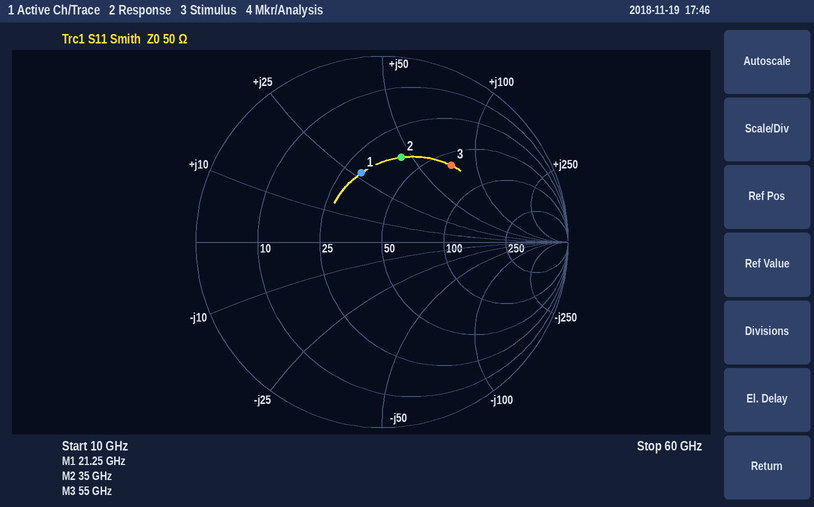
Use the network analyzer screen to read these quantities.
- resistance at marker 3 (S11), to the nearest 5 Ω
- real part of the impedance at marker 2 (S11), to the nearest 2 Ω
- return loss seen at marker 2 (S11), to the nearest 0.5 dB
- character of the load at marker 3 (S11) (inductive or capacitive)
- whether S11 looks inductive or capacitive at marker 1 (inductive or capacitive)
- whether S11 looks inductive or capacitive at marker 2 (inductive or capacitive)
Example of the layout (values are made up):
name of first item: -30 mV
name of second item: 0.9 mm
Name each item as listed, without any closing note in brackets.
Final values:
resistance at marker 3 (S11), to the nearest 5 Ω: 60 Ω
real part of the impedance at marker 2 (S11), to the nearest 2 Ω: 38 Ω
return loss seen at marker 2 (S11), to the nearest 0.5 dB: 6.5 dB
character of the load at marker 3 (S11): inductive
whether S11 looks inductive or capacitive at marker 1: inductive
whether S11 looks inductive or capacitive at marker 2: inductive
